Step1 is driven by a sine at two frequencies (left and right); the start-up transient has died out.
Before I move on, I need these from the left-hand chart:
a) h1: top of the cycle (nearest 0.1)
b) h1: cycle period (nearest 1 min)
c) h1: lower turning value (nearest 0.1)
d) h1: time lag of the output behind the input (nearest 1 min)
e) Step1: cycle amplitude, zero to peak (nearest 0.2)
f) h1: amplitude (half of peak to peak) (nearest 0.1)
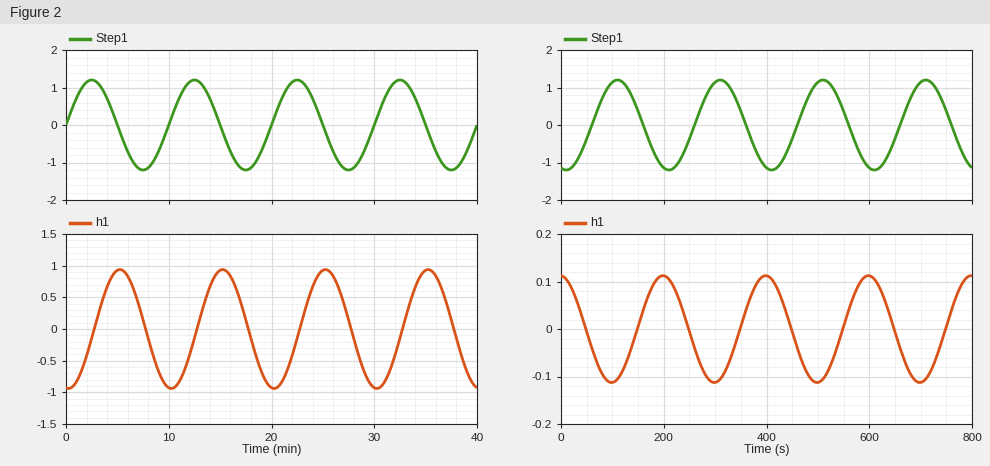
0.9
10 min
-0.9
3 min
1.2
0.9
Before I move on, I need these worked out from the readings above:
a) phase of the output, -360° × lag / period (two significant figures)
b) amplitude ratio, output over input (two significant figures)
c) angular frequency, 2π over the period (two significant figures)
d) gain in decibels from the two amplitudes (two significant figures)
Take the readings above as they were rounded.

-110°
0.75
0.63 rad/min
-2.5 dB
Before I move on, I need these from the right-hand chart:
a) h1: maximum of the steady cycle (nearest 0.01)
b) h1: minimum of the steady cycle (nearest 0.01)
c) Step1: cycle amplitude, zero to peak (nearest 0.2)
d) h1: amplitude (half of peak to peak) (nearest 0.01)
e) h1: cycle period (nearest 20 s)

0.11
-0.11
1.2
0.11
200 s
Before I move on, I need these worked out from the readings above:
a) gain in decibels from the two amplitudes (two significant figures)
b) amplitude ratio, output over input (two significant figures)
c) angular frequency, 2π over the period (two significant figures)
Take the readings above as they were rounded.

-21 dB
0.092
0.031 rad/s
